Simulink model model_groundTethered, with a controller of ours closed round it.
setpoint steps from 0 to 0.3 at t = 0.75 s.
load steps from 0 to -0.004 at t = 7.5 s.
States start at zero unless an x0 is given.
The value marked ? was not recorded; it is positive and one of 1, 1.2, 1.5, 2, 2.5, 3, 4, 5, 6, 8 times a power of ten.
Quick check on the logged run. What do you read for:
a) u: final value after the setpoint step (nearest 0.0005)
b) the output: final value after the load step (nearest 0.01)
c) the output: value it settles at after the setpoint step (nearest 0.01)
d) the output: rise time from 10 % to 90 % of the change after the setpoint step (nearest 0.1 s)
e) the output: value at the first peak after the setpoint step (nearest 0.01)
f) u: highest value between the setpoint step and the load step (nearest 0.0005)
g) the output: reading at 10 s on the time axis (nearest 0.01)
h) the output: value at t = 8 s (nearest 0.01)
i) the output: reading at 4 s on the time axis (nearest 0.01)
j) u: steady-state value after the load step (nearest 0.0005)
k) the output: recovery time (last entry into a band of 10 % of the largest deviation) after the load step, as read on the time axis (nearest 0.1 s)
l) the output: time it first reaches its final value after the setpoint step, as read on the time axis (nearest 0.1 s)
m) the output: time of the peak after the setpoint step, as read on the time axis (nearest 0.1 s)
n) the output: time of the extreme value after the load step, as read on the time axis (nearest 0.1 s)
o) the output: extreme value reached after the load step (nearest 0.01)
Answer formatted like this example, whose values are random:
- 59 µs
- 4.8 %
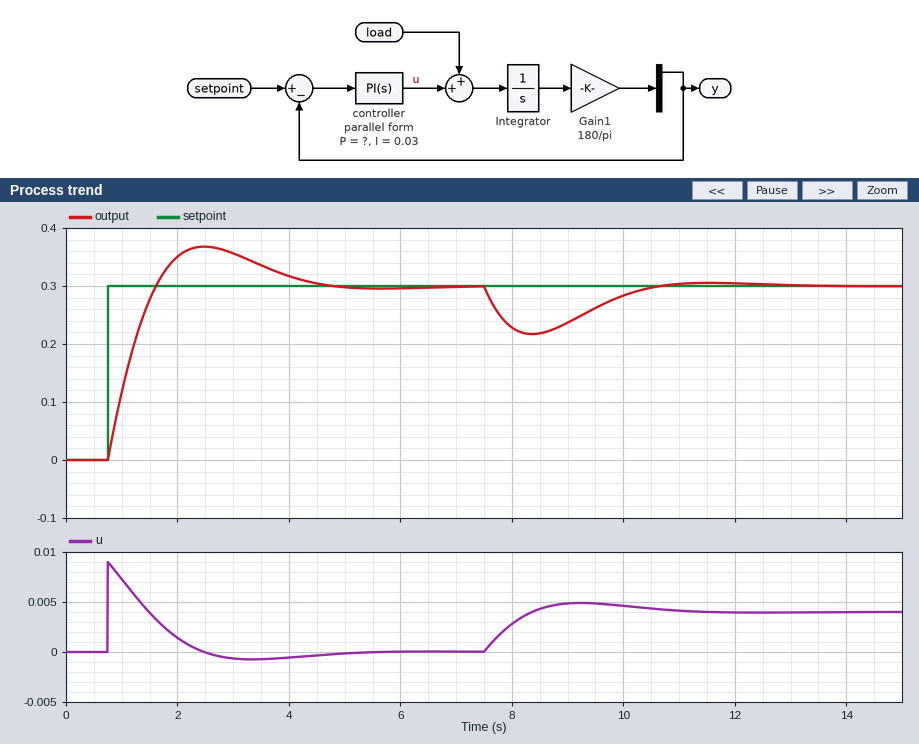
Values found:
- 0.0000
- 0.30
- 0.30
- 0.7 s
- 0.37
- 0.0090
- 0.28
- 0.23
- 0.32
- 0.0040
- 10.3 s
- 1.6 s
- 2.5 s
- 8.4 s
- 0.22
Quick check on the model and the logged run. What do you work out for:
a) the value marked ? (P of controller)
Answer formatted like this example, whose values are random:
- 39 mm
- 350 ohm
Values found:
- 0.03
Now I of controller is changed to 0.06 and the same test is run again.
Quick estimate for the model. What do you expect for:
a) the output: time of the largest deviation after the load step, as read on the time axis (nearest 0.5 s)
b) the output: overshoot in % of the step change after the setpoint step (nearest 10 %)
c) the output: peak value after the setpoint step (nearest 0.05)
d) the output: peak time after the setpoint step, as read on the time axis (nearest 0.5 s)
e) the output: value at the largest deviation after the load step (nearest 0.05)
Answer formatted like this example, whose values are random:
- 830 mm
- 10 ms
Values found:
- 8.0 s
- 30 %
- 0.40
- 2.0 s
- 0.25
